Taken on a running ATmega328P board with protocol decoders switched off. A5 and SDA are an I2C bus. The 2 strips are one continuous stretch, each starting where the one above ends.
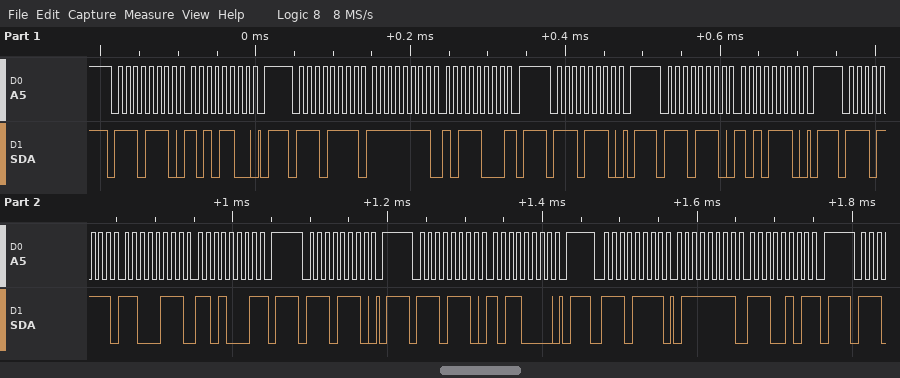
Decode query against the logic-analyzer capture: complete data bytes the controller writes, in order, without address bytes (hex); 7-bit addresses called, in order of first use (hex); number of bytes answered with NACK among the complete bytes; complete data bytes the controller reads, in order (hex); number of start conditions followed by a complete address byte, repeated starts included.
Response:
AC AE B0
0x77
3
FF B8 C7 D1 7F E5
8
